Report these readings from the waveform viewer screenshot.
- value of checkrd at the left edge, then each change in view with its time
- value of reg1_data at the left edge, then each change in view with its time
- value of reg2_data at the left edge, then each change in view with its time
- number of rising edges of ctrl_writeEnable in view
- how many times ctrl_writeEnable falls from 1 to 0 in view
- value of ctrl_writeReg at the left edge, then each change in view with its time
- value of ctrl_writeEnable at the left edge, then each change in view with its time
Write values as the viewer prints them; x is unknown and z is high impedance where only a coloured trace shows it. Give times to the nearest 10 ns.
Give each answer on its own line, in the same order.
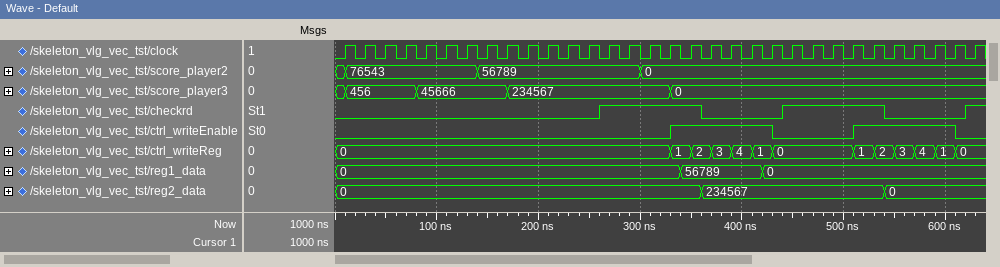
0, 1 at 260 ns, 0 at 360 ns, 1 at 440 ns, 0 at 540 ns, 1 at 620 ns
0, 56789 at 340 ns, 0 at 420 ns
0, 234567 at 360 ns, 0 at 540 ns
2
2
0, 1 at 330 ns, 2 at 350 ns, 3 at 370 ns, 4 at 390 ns, 1 at 410 ns, 0 at 430 ns, 1 at 510 ns, 2 at 530 ns, 3 at 550 ns, 4 at 570 ns, 1 at 590 ns, 0 at 610 ns
0, 1 at 330 ns, 0 at 430 ns, 1 at 510 ns, 0 at 610 ns
